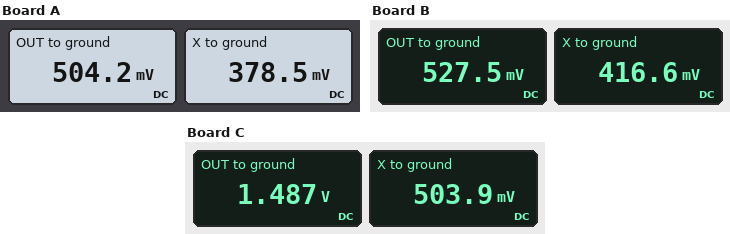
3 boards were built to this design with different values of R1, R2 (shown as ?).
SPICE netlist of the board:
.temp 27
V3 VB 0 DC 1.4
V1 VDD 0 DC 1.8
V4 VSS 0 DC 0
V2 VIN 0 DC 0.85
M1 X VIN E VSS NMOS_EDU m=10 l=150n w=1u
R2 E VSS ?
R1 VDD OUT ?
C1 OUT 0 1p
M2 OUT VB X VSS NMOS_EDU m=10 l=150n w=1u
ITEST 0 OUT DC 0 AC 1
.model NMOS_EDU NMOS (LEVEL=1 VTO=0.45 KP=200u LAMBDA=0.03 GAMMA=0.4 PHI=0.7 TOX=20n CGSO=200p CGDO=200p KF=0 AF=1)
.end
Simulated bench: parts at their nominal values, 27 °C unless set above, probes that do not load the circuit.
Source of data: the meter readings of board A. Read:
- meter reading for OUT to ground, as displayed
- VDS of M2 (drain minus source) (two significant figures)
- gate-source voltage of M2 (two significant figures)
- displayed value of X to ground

504.2 mV
130 mV
1.0 V
378.5 mV
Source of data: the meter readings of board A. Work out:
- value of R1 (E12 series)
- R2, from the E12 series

1.8 kΩ
82 Ω
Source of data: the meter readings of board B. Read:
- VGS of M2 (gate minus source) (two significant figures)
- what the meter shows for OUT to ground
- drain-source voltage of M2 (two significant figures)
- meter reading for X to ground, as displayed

980 mV
527.5 mV
110 mV
416.6 mV
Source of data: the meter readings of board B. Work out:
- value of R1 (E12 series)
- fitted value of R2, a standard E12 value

2.2 kΩ
150 Ω
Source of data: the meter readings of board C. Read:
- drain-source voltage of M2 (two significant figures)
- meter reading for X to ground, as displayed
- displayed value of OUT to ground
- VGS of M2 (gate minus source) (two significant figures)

980 mV
503.9 mV
1.487 V
900 mV
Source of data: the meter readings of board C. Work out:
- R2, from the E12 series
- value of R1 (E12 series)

56 Ω
390 Ω
